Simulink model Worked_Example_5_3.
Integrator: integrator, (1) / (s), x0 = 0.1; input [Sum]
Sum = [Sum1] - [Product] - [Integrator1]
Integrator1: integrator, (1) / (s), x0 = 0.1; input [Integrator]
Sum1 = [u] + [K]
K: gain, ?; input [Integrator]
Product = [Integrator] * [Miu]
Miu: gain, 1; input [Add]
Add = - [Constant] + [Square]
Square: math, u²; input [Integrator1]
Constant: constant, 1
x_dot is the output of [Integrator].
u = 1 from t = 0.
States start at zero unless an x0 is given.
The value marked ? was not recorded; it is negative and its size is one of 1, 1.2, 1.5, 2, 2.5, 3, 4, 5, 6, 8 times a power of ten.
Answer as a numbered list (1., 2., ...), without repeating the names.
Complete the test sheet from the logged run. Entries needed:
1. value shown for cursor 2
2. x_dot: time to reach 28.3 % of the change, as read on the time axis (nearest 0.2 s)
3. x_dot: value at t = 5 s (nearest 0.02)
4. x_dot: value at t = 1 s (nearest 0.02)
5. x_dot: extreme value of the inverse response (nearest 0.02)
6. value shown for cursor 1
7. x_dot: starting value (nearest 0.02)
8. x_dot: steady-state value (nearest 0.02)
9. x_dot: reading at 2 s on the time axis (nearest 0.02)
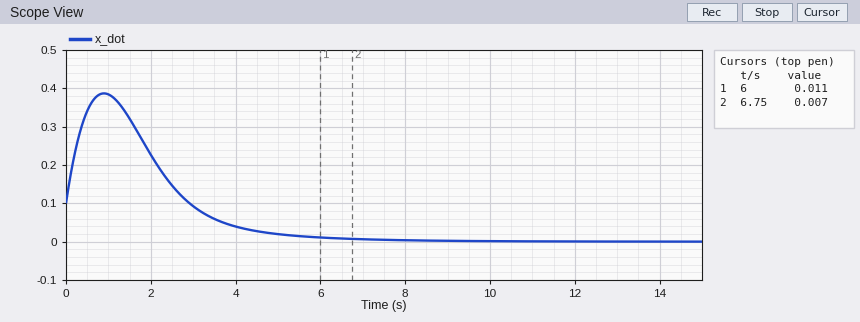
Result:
1. 0.007
2. 3.2 s
3. 0.02
4. 0.38
5. 0.38
6. 0.011
7. 0.10
8. 0.00
9. 0.22
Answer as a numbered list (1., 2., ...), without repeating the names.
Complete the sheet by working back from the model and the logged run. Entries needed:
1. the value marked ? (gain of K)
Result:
1. -2.5
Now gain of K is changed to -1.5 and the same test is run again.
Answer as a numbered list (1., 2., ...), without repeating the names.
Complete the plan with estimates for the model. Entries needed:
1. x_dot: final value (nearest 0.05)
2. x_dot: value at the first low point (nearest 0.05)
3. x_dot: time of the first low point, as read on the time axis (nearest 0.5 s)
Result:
1. 0.00
2. -0.05
3. 4.0 s
